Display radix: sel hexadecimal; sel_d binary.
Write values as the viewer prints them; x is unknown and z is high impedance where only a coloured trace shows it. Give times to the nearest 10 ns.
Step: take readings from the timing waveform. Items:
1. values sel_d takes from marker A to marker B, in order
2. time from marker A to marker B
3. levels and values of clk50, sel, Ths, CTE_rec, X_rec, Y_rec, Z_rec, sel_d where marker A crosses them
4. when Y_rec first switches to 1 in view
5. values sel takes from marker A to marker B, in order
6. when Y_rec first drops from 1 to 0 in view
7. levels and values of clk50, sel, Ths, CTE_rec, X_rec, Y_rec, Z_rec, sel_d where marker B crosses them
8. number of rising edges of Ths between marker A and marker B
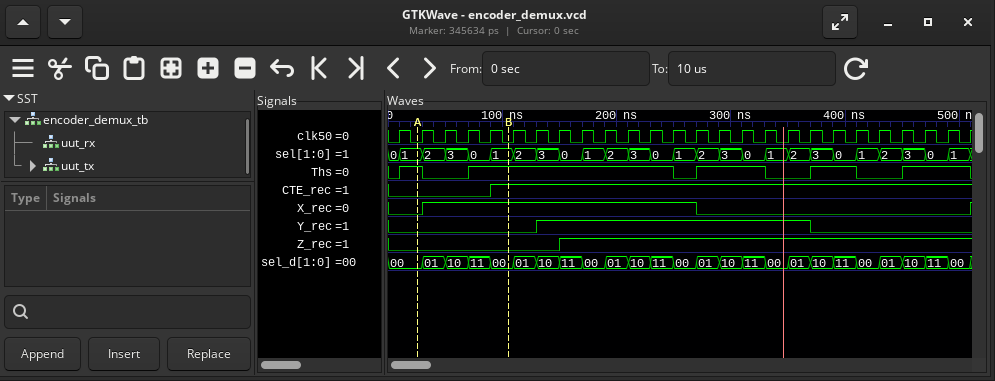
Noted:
00, 01, 10, 11, 00
80 ns
clk50=0, sel=1, Ths=1, CTE_rec=0, X_rec=0, Y_rec=0, Z_rec=0, sel_d=00
130 ns
1, 2, 3, 0, 1
370 ns
clk50=0, sel=1, Ths=1, CTE_rec=1, X_rec=1, Y_rec=0, Z_rec=0, sel_d=00
1
